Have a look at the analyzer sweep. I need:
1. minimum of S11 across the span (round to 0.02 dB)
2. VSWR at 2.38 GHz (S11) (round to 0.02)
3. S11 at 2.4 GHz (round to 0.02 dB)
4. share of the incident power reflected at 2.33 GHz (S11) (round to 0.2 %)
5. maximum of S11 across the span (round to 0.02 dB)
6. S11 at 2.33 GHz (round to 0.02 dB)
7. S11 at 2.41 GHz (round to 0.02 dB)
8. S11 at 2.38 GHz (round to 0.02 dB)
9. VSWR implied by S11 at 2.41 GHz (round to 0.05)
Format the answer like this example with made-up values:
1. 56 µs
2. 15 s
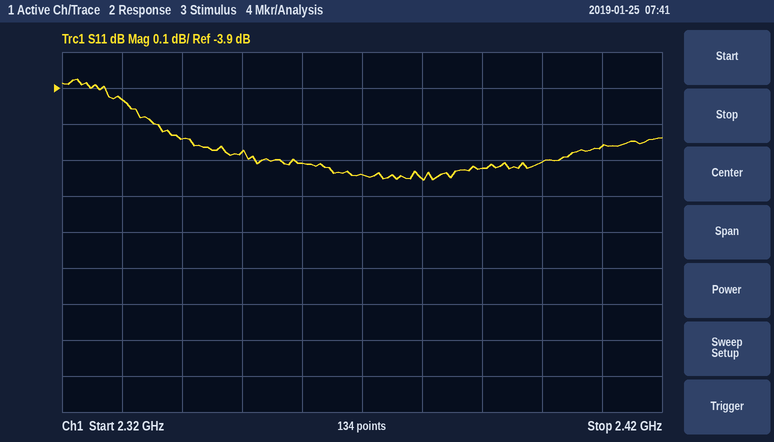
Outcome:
1. -4.16 dB
2. 4.26
3. -4.10 dB
4. 40.4 %
5. -3.88 dB
6. -3.94 dB
7. -4.06 dB
8. -4.16 dB
9. 4.35
